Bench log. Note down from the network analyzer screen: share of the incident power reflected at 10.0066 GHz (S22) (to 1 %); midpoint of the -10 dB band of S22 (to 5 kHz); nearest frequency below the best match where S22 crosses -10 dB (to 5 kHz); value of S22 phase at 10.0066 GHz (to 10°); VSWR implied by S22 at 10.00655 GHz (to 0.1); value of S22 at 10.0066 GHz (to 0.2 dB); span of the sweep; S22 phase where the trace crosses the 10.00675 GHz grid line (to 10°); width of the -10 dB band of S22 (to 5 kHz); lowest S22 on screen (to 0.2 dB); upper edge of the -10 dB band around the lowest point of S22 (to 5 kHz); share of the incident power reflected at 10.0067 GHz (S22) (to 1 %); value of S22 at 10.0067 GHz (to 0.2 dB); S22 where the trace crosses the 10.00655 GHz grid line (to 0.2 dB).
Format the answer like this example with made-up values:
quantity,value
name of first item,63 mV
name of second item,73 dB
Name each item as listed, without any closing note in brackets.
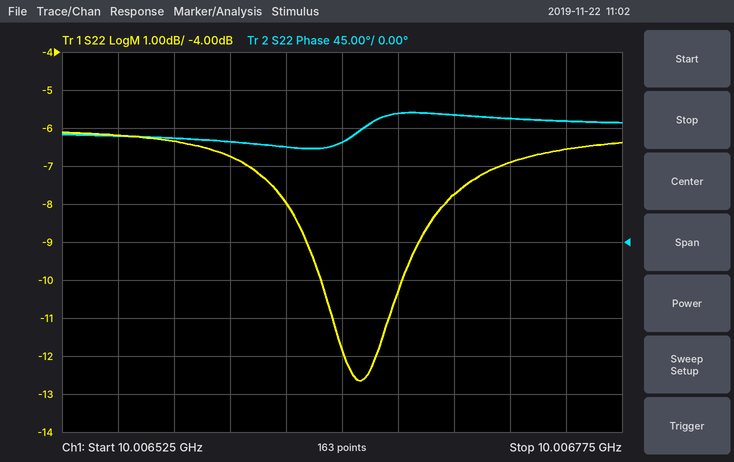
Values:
quantity,value
share of the incident power reflected at 10.0066 GHz (S22),21 %
midpoint of the -10 dB band of S22,10.006660 GHz
nearest frequency below the best match where S22 crosses -10 dB,10.006640 GHz
value of S22 phase at 10.0066 GHz,120°
VSWR implied by S22 at 10.00655 GHz,2.9
value of S22 at 10.0066 GHz,-6.8 dB
span of the sweep,250 kHz
S22 phase where the trace crosses the 10.00675 GHz grid line,140°
width of the -10 dB band of S22,35 kHz
lowest S22 on screen,-12.6 dB
upper edge of the -10 dB band around the lowest point of S22,10.006675 GHz
share of the incident power reflected at 10.0067 GHz (S22),17 %
value of S22 at 10.0067 GHz,-7.8 dB
S22 where the trace crosses the 10.00655 GHz grid line,-6.2 dB
